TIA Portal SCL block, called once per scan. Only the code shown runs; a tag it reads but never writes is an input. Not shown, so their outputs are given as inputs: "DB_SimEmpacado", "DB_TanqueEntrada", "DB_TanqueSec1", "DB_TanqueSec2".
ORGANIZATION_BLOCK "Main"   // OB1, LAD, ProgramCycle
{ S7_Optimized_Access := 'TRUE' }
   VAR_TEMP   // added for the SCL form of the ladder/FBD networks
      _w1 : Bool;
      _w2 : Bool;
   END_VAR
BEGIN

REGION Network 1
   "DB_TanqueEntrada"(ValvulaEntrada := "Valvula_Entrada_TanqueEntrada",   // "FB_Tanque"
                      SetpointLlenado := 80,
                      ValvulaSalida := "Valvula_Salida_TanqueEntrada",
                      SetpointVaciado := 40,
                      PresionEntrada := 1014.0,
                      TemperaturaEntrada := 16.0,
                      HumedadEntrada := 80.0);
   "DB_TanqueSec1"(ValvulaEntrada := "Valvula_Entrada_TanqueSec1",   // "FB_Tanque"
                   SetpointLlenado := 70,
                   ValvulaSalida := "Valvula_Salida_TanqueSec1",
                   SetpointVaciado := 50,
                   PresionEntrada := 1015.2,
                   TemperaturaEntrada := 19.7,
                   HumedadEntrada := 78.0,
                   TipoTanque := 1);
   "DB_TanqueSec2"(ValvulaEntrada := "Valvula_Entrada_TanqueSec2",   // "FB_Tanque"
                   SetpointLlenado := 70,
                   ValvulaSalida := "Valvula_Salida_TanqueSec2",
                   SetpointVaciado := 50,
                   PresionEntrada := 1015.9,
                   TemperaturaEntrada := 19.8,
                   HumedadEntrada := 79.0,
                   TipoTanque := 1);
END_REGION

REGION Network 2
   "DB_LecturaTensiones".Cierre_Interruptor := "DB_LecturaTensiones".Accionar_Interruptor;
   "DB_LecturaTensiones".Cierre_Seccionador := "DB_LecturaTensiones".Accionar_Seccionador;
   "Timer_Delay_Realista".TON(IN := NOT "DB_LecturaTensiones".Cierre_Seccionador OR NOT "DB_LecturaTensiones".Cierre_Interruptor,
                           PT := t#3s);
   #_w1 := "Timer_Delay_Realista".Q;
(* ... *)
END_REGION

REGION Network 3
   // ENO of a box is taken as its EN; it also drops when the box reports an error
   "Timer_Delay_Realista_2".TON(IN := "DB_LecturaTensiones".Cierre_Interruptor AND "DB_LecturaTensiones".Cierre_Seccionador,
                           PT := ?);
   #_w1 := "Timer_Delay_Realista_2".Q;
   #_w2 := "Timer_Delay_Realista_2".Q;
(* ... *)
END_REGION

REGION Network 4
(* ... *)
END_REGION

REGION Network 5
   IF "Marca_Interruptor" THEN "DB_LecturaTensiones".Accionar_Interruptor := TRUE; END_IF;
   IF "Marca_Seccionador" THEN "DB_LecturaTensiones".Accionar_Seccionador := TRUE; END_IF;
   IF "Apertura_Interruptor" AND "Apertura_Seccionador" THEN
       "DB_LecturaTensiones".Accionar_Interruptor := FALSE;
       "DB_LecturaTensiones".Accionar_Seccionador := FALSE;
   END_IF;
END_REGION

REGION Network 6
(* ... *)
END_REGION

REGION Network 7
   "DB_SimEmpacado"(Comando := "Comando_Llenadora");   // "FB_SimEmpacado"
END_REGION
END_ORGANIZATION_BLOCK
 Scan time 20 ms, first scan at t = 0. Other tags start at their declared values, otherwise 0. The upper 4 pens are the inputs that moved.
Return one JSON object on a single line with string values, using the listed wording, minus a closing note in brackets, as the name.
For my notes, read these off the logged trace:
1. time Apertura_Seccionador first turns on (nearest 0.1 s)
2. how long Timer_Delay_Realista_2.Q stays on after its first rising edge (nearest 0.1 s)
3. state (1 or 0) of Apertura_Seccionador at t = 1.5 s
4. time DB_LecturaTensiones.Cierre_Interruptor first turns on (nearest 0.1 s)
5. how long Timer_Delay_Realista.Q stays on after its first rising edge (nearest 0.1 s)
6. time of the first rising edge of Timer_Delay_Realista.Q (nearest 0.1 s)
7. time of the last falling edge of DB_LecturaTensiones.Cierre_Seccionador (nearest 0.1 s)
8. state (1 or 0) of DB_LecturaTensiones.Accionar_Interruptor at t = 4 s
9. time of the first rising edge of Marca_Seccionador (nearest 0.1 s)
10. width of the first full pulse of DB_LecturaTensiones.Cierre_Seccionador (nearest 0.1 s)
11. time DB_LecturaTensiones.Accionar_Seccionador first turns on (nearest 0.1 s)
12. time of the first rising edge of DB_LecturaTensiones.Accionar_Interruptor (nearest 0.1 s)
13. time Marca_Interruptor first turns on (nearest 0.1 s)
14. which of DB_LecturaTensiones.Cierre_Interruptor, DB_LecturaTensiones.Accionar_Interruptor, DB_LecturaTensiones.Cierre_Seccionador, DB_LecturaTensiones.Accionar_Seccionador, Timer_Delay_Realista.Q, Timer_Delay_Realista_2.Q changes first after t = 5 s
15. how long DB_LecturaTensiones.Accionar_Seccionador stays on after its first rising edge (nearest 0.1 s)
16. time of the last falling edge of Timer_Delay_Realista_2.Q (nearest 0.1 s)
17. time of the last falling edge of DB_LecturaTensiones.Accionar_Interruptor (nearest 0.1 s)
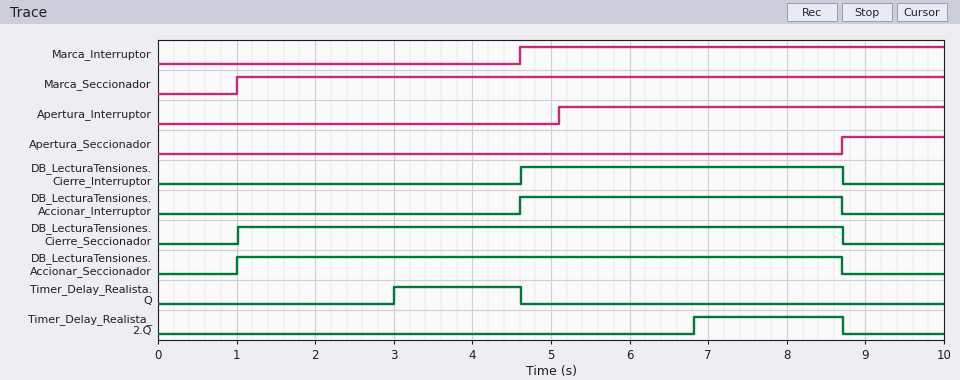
{"time Apertura_Seccionador first turns on": "8.7 s", "how long Timer_Delay_Realista_2.Q stays on after its first rising edge": "1.9 s", "state (1 or 0) of Apertura_Seccionador at t = 1.5 s": "0", "time DB_LecturaTensiones.Cierre_Interruptor first turns on": "4.6 s", "how long Timer_Delay_Realista.Q stays on after its first rising edge": "1.6 s", "time of the first rising edge of Timer_Delay_Realista.Q": "3.0 s", "time of the last falling edge of DB_LecturaTensiones.Cierre_Seccionador": "8.7 s", "state (1 or 0) of DB_LecturaTensiones.Accionar_Interruptor at t = 4 s": "0", "time of the first rising edge of Marca_Seccionador": "1.0 s", "width of the first full pulse of DB_LecturaTensiones.Cierre_Seccionador": "7.7 s", "time DB_LecturaTensiones.Accionar_Seccionador first turns on": "1.0 s", "time of the first rising edge of DB_LecturaTensiones.Accionar_Interruptor": "4.6 s", "time Marca_Interruptor first turns on": "4.6 s", "which of DB_LecturaTensiones.Cierre_Interruptor, DB_LecturaTensiones.Accionar_Interruptor, DB_LecturaTensiones.Cierre_Seccionador, DB_LecturaTensiones.Accionar_Seccionador, Timer_Delay_Realista.Q, Timer_Delay_Realista_2.Q changes first after t = 5 s": "Timer_Delay_Realista_2.Q", "how long DB_LecturaTensiones.Accionar_Seccionador stays on after its first rising edge": "7.7 s", "time of the last falling edge of Timer_Delay_Realista_2.Q": "8.7 s", "time of the last falling edge of DB_LecturaTensiones.Accionar_Interruptor": "8.7 s"}
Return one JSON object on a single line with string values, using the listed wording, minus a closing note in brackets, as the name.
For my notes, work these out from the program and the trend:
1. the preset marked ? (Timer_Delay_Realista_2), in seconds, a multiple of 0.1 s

{"the preset marked ? (Timer_Delay_Realista_2), in seconds, a multiple of 0.1 s": "2.2 s"}
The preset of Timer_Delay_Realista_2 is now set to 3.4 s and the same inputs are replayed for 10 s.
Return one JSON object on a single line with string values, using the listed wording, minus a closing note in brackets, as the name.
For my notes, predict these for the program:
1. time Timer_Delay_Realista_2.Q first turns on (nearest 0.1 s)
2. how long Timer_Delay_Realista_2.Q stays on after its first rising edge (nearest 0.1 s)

{"time Timer_Delay_Realista_2.Q first turns on": "8.0 s", "how long Timer_Delay_Realista_2.Q stays on after its first rising edge": "0.7 s"}
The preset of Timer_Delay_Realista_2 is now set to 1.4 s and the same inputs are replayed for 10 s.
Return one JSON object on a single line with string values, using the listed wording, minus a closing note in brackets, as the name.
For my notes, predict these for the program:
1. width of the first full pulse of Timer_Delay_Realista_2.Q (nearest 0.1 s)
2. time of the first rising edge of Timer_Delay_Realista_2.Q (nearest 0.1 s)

{"width of the first full pulse of Timer_Delay_Realista_2.Q": "2.7 s", "time of the first rising edge of Timer_Delay_Realista_2.Q": "6.0 s"}
